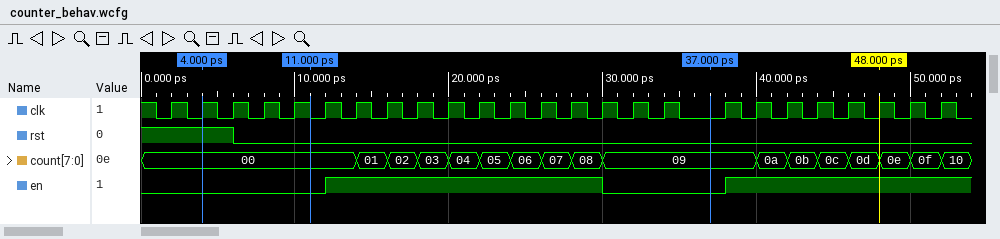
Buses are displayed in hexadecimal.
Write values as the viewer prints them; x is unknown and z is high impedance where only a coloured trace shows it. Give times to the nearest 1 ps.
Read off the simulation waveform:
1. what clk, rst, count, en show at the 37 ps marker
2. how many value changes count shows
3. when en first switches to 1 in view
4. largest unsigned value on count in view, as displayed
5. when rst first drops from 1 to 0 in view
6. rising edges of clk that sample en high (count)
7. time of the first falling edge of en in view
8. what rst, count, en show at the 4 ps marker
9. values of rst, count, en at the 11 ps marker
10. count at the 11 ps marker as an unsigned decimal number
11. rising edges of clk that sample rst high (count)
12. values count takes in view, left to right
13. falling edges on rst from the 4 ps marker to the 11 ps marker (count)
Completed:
clk=0, rst=0, count=09, en=0
16
12 ps
10
6 ps
16
30 ps
rst=1, count=00, en=0
rst=0, count=00, en=0
0
3
00, 01, 02, 03, 04, 05, 06, 07, 08, 09, 0a, 0b, 0c, 0d, 0e, 0f, 10
1
